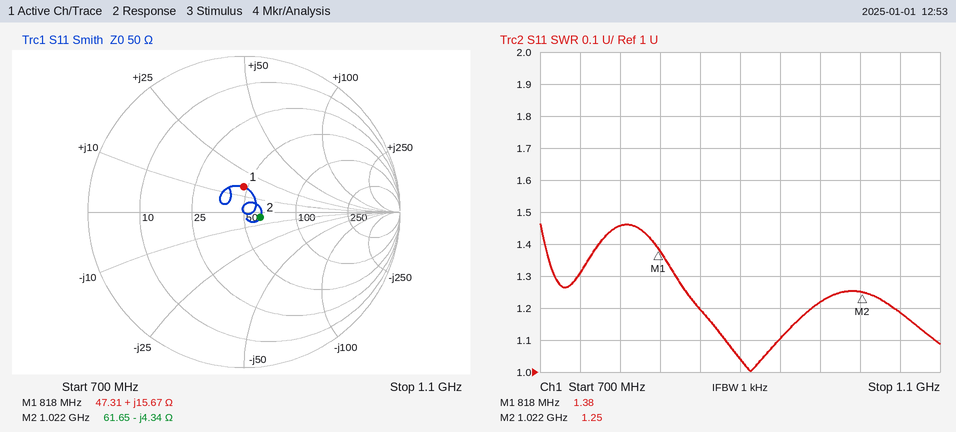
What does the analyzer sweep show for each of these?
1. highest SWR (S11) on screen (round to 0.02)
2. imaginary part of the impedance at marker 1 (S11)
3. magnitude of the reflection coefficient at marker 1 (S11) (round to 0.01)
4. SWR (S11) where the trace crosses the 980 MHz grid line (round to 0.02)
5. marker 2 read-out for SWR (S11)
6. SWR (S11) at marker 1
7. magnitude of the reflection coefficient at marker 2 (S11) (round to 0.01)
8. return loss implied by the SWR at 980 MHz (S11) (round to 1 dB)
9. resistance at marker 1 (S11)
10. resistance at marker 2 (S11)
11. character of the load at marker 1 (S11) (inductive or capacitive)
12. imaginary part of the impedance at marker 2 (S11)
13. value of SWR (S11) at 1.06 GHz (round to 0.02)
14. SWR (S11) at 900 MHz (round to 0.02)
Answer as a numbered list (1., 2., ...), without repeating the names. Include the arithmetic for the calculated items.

1. 1.46
2. +15.67 Ω
3. 0.16
4. 1.22
5. 1.25
6. 1.38
7. 0.11
8. −20 log10((1.22 − 1)/(1.22 + 1)) ≈ 20 dB
9. 47.31 Ω
10. 61.65 Ω
11. inductive
12. -4.34 Ω
13. 1.18
14. 1.04
